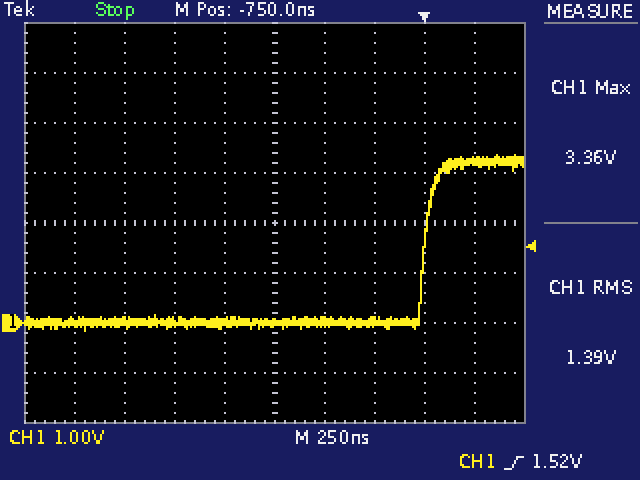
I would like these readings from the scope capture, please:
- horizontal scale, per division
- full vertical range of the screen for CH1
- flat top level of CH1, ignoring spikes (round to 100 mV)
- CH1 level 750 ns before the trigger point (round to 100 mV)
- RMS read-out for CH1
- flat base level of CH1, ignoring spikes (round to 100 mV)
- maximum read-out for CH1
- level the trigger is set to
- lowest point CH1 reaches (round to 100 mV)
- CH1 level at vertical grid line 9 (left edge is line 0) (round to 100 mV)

250 ns
8 V
3.2 V
0.0 V
1.39 V
0.0 V
3.36 V
1.52 V
-200 mV
3.2 V
